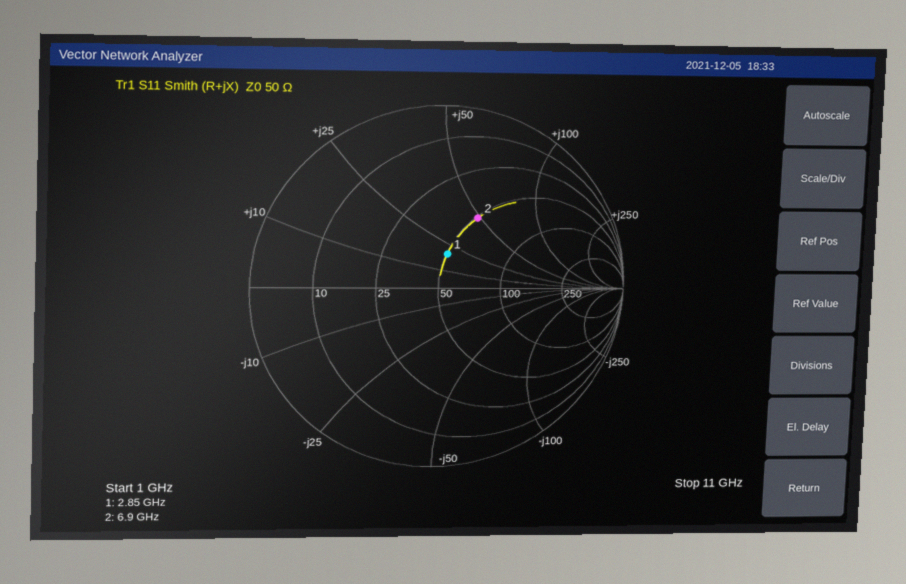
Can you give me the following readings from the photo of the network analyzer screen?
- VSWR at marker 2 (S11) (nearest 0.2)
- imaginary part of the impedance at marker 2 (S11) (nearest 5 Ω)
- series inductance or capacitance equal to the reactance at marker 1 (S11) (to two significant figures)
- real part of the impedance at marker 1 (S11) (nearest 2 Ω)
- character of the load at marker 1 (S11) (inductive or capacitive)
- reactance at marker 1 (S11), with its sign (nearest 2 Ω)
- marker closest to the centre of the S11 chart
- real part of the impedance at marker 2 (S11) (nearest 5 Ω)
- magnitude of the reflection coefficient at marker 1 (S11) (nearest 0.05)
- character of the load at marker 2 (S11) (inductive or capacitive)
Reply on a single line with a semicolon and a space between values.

2.6; +50 Ω; 1.1 nH; 50 Ω; inductive; +20 Ω; marker 1; 50 Ω; 0.20; inductive
